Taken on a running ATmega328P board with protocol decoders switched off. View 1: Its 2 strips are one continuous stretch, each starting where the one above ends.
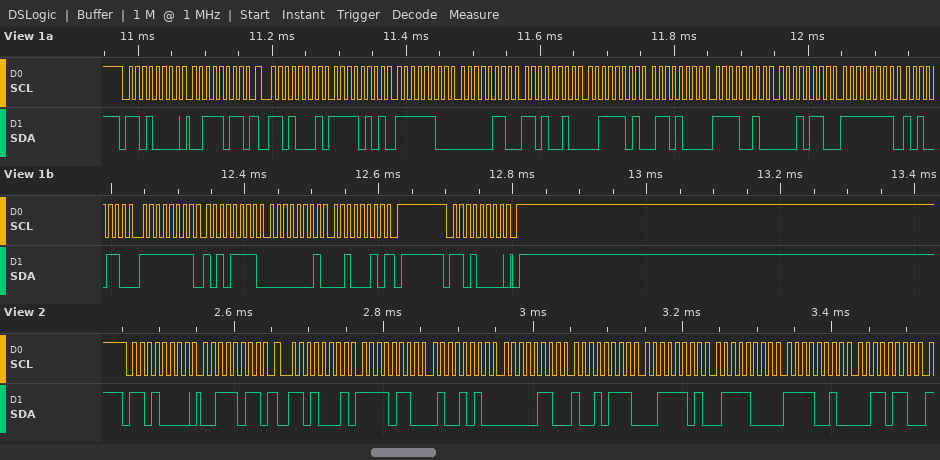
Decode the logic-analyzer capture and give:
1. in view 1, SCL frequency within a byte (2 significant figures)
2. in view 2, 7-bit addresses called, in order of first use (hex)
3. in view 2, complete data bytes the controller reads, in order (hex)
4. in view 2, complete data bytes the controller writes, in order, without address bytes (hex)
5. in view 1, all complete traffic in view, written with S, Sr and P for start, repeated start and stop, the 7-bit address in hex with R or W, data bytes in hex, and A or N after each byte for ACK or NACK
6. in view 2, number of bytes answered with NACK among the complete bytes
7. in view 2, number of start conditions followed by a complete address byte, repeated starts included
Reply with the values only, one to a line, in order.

100 kHz
0x68
F6 4A 06 97 3D 78 F2 36
3B
S 68W A 3B A Sr 68R A F5 A FC A 06 A D2 A 3D A 68 A F2 A 16 A FF A A6 A FF A AF A 01 A 22 N P S 68W A P
0
2
